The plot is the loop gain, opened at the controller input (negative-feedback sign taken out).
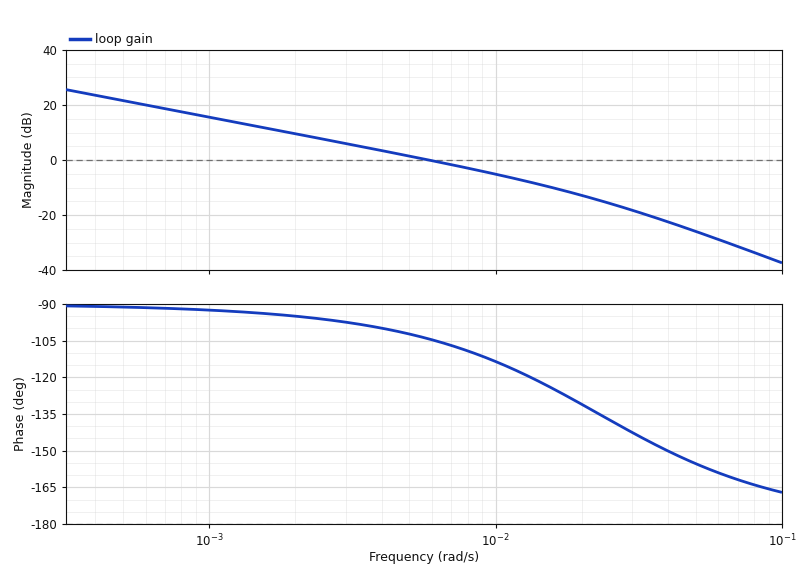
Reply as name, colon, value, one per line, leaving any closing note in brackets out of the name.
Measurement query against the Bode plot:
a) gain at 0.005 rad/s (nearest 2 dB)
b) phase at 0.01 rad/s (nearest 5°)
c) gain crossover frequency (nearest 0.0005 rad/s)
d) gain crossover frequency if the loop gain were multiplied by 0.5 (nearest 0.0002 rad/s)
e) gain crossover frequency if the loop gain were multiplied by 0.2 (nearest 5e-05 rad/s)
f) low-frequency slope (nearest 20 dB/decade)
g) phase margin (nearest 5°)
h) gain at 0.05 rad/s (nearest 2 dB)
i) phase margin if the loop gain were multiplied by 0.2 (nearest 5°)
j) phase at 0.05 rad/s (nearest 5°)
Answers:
gain at 0.005 rad/s: 2 dB
phase at 0.01 rad/s: -115°
gain crossover frequency: 0.0060 rad/s
gain crossover frequency if the loop gain were multiplied by 0.5: 0.0030 rad/s
gain crossover frequency if the loop gain were multiplied by 0.2: 0.00120 rad/s
low-frequency slope: -20 dB/decade
phase margin: 75°
gain at 0.05 rad/s: -26 dB
phase margin if the loop gain were multiplied by 0.2: 85°
phase at 0.05 rad/s: -155°
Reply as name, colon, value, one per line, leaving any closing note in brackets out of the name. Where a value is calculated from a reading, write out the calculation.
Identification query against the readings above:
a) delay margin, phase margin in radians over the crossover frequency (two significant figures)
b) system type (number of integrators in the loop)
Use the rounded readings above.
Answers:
delay margin, phase margin in radians over the crossover frequency: 75 × π / 180 / 0.006 = 220 s
system type: 1
